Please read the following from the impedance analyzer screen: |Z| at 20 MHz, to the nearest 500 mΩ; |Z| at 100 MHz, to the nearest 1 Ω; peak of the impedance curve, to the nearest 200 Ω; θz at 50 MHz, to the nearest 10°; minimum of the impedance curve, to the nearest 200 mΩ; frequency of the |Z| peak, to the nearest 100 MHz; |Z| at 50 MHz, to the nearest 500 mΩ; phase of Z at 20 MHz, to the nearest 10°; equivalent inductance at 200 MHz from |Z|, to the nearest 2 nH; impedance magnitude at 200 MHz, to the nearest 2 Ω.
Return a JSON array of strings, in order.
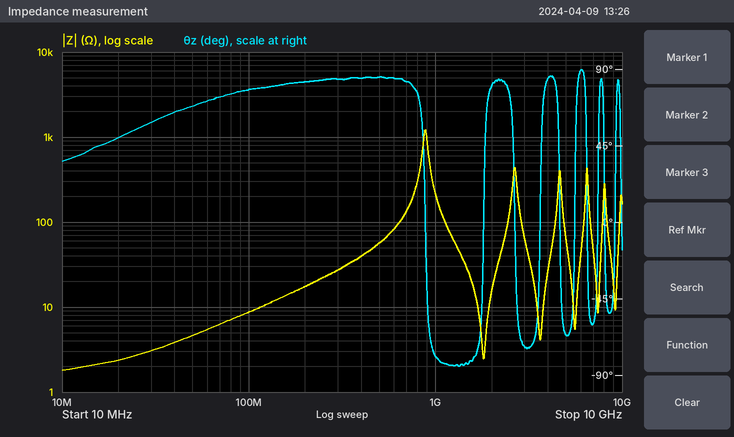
["2.5 Ω", "9 Ω", "1.2 kΩ", "70°", "1.8 Ω", "900 MHz", "4.5 Ω", "50°", "14 nH", "18 Ω"]
